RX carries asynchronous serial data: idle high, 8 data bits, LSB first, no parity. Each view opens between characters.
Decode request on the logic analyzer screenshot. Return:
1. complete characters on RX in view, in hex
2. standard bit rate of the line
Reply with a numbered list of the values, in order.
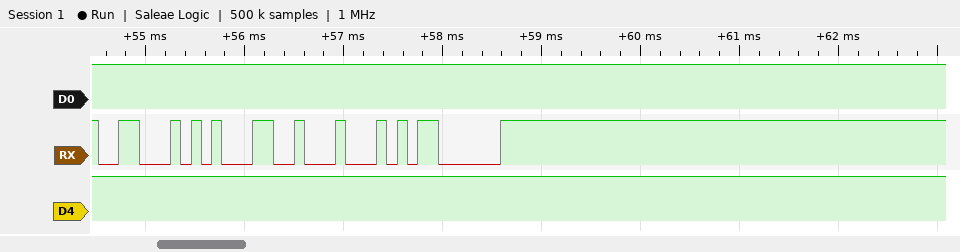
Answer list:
1. 46, 31, 44, 03
2. 9600 baud
